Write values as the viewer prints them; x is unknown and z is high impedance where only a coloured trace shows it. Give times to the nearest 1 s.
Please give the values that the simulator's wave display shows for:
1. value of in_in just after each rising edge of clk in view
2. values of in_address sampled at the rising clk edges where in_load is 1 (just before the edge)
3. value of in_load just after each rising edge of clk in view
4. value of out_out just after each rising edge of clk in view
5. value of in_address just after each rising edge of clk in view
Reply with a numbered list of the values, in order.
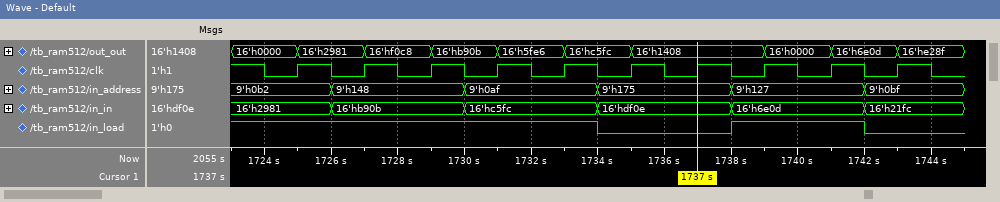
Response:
1. 16'h2981, 16'hb90b, 16'hb90b, 16'hc5fc, 16'hc5fc, 16'hdf0e, 16'hdf0e, 16'h6e0d, 16'h6e0d, 16'h21fc
2. 9'h0b2, 9'h148, 9'h148, 9'h0af, 9'h0af, 9'h127, 9'h127
3. 1 1 1 1 1 0 0 1 1 0
4. 16'h2981, 16'hf0c8, 16'hb90b, 16'h5fe6, 16'hc5fc, 16'h1408, 16'h1408, 16'h0000, 16'h6e0d, 16'he28f
5. 9'h0b2, 9'h148, 9'h148, 9'h0af, 9'h0af, 9'h175, 9'h175, 9'h127, 9'h127, 9'h0bf
